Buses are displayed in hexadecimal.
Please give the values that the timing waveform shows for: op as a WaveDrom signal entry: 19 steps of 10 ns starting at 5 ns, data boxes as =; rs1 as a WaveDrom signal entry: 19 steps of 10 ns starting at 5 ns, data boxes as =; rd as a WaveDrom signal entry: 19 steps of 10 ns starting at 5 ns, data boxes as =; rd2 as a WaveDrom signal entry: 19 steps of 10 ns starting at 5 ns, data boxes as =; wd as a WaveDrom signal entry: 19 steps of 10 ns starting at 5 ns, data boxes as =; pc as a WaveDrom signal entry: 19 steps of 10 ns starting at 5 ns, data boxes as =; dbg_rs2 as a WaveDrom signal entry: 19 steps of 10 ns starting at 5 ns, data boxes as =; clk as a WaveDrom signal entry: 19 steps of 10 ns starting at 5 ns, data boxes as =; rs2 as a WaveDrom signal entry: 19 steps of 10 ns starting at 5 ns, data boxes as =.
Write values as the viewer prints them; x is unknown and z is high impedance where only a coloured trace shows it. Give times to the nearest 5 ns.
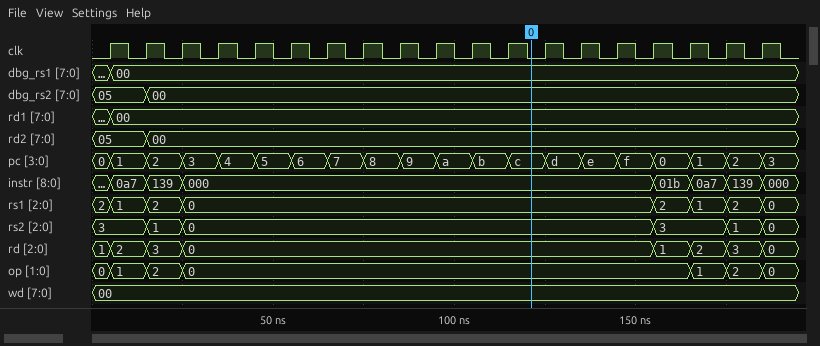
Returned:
{name: 'op', wave: '===.............===', data: '1 2 0 1 2 0'}
{name: 'rs1', wave: '===............====', data: '1 2 0 2 1 2 0'}
{name: 'rd', wave: '===............====', data: '2 3 0 1 2 3 0'}
{name: 'rd2', wave: '==.................', data: '05 00'}
{name: 'wd', wave: '=..................', data: '00'}
{name: 'pc', wave: '===================', data: '1 2 3 4 5 6 7 8 9 a b c d e f 0 1 2 3'}
{name: 'dbg_rs2', wave: '==.................', data: '05 00'}
{name: 'clk', wave: 'p..................'}
{name: 'rs2', wave: '===............=.==', data: '3 1 0 3 1 0'}
